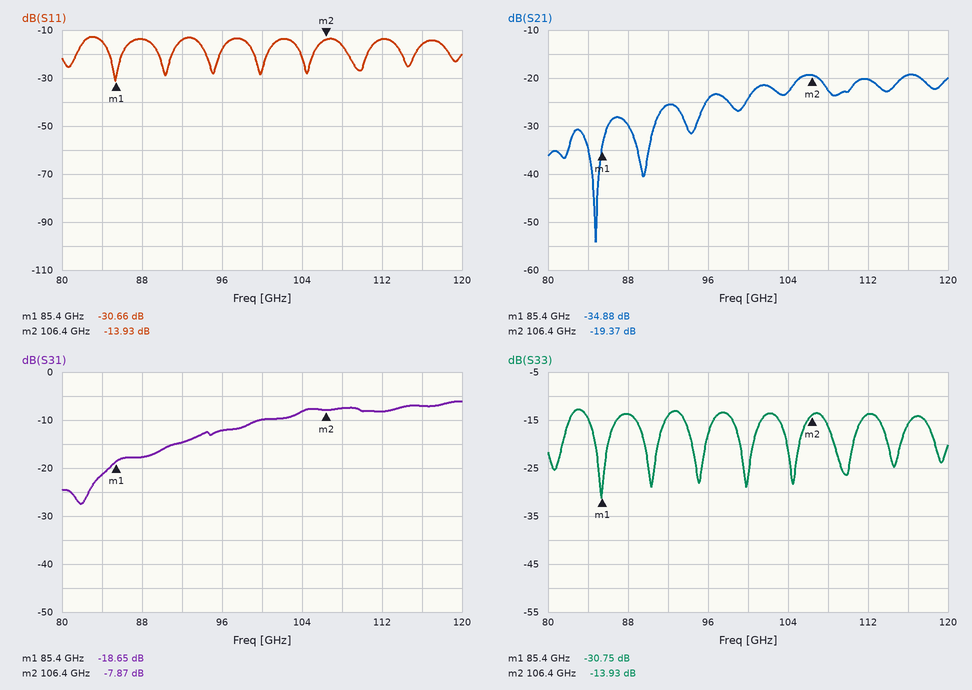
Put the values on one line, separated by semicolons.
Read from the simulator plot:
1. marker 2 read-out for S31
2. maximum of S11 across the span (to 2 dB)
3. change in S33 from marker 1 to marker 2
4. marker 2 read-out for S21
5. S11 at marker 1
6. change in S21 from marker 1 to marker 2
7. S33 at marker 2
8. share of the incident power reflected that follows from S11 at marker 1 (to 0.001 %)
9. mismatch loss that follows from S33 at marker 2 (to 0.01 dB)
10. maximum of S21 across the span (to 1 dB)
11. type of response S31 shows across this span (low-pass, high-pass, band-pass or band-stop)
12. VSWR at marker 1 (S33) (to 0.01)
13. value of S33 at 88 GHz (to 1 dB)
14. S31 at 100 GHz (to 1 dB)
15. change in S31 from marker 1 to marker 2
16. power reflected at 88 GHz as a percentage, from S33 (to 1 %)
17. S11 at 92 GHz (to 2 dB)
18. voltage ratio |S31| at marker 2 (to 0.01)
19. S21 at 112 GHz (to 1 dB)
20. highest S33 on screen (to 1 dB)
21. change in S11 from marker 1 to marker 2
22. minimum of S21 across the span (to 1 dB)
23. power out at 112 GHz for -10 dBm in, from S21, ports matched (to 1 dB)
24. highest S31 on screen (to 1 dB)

-7.87 dB; -12 dB; 16.82 dB; -19.37 dB; -30.66 dB; 15.51 dB; -13.93 dB; 0.086 %; 0.18 dB; -19 dB; high-pass; 1.06; -14 dB; -10 dB; 10.78 dB; 4 %; -14 dB; 0.40; -20 dB; -13 dB; 16.73 dB; -54 dB; -30 dBm; -6 dB
